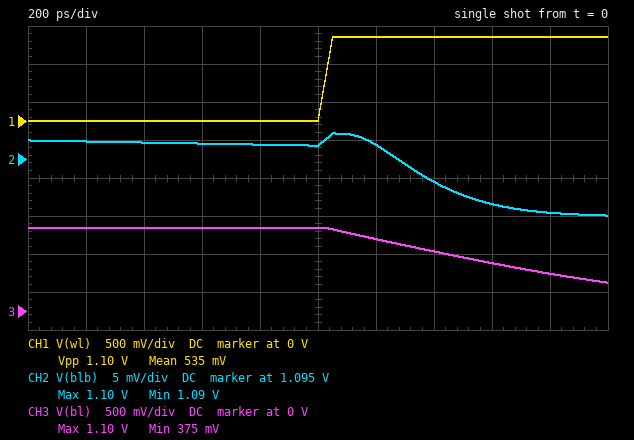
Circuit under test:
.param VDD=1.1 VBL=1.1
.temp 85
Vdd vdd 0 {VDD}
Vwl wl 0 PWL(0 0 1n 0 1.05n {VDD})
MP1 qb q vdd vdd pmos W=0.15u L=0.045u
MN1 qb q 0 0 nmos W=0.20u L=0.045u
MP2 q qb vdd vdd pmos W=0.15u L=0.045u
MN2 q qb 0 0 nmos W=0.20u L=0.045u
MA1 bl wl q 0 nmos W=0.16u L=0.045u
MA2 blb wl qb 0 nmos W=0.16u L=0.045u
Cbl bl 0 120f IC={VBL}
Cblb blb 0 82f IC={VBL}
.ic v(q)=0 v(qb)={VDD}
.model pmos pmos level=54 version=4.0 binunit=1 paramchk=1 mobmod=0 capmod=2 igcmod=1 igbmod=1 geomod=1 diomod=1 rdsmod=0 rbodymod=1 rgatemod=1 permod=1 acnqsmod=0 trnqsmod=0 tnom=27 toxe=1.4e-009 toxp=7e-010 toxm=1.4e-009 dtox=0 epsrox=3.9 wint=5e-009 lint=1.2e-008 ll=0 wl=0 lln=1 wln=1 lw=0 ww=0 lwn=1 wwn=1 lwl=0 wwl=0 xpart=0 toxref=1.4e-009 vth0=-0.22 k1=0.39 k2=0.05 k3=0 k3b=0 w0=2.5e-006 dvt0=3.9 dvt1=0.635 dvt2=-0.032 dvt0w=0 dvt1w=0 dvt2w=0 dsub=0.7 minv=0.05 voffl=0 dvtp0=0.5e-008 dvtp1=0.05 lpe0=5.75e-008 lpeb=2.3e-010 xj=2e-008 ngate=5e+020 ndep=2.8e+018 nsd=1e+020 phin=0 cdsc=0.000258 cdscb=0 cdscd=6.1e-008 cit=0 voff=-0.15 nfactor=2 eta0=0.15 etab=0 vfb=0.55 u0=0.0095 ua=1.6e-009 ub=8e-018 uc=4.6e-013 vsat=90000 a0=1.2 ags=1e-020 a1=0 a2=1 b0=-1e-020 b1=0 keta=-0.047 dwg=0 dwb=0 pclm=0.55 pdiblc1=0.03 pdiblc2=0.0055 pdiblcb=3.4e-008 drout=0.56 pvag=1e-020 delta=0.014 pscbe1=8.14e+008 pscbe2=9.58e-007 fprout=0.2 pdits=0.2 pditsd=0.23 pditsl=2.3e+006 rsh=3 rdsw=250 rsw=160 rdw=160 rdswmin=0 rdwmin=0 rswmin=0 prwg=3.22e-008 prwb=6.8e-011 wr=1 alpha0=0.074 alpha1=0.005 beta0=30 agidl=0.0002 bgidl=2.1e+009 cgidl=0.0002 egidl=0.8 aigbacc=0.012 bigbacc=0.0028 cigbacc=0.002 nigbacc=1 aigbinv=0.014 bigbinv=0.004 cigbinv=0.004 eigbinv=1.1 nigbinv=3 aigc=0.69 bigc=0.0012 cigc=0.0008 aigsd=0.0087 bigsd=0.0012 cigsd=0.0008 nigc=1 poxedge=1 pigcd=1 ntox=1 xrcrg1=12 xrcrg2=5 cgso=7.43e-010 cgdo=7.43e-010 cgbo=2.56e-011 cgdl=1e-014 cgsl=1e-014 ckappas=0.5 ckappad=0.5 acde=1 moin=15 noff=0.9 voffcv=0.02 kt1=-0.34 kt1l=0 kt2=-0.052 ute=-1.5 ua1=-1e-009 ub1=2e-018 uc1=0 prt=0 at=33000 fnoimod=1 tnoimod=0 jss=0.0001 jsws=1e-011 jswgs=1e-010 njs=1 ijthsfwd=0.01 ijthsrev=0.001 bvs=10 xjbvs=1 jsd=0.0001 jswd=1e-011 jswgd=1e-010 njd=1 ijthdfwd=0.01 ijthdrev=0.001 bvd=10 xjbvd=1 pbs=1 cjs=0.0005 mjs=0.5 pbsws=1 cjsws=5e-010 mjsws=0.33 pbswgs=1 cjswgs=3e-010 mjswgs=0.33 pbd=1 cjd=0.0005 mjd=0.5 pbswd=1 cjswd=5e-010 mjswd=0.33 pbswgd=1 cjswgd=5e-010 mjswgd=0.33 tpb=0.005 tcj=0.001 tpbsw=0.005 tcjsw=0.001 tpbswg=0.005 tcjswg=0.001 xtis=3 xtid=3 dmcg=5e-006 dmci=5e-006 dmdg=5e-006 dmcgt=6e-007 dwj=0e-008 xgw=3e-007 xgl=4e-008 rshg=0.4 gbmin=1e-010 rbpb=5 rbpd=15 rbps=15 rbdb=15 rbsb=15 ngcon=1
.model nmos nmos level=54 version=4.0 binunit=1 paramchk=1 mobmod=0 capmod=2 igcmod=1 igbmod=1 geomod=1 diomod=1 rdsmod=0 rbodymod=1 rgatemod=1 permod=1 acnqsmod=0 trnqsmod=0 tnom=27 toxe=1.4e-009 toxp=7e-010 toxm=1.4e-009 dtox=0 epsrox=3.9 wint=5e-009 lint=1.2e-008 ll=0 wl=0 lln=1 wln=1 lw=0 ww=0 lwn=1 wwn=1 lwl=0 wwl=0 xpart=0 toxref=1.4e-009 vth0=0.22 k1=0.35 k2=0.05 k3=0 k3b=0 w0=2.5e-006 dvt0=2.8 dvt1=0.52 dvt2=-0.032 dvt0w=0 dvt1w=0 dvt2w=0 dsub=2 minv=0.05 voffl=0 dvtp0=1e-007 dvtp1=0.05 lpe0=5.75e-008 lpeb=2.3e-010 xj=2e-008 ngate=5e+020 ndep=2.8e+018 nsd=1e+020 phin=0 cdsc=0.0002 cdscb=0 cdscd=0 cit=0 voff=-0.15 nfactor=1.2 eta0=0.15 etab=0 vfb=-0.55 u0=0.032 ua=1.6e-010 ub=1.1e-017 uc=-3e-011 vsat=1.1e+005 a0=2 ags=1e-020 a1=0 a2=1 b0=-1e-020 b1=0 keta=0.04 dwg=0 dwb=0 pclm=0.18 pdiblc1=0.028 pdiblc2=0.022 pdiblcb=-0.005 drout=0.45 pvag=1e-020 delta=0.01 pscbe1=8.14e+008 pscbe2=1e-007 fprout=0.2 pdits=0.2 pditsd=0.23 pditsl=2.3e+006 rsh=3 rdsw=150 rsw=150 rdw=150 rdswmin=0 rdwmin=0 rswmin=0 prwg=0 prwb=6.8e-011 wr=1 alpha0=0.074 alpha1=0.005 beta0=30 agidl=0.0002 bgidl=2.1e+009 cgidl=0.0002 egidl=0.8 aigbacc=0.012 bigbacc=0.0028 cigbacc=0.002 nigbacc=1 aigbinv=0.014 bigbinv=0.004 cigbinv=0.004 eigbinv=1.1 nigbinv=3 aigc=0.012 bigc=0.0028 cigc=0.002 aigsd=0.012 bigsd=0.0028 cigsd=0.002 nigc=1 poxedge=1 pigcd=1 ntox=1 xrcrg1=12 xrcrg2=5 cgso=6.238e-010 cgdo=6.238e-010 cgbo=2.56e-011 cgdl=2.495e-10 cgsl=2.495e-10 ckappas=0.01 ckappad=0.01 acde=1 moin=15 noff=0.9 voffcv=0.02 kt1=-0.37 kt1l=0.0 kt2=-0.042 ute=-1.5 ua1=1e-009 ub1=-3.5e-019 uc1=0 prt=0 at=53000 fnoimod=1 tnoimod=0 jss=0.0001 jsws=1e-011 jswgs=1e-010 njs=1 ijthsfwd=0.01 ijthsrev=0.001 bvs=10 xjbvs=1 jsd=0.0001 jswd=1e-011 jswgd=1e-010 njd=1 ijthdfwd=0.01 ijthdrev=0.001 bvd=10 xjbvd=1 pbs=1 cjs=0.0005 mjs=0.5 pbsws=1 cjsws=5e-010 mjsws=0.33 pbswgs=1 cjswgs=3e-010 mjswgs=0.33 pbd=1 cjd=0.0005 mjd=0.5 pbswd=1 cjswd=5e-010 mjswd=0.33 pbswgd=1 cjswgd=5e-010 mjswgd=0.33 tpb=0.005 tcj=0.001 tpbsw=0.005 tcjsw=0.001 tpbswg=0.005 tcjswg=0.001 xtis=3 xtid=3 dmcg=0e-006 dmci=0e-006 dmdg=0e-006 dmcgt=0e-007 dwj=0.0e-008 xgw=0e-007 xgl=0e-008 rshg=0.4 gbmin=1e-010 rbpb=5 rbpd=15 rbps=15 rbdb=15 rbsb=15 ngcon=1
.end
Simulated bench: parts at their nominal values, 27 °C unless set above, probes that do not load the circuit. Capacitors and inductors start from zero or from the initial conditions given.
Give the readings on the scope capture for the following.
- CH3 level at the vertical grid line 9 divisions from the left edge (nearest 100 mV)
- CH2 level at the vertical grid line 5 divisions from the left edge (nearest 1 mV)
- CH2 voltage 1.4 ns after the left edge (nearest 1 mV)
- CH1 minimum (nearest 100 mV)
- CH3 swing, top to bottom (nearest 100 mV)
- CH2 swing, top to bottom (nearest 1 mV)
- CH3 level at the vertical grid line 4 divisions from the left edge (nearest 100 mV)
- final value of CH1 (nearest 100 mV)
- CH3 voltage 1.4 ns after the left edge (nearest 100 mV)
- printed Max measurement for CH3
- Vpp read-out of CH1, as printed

500 mV
1.097 V
1.092 V
0 V
700 mV
11 mV
1.1 V
1.1 V
800 mV
1.10 V
1.10 V
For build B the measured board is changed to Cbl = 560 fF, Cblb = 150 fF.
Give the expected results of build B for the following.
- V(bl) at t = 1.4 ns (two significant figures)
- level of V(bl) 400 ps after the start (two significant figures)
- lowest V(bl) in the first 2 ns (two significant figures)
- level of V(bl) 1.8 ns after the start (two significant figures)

1.0 V
1.1 V
920 mV
960 mV
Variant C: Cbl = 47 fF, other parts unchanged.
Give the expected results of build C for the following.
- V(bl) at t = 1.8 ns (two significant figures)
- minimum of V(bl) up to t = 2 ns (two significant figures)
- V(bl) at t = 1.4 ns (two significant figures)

80 mV
35 mV
380 mV
